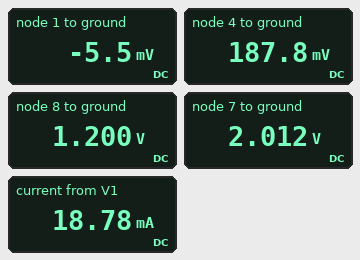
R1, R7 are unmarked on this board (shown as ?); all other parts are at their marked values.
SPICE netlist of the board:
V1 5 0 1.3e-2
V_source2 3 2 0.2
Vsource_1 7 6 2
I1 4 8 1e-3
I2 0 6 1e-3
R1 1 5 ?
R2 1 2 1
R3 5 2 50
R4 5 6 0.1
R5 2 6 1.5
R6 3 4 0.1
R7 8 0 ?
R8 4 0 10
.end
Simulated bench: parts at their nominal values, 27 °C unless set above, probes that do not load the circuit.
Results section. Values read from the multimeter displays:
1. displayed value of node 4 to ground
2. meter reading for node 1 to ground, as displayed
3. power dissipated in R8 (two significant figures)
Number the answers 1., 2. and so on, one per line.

1. 187.8 mV
2. -5.5 mV
3. 3.5 mW
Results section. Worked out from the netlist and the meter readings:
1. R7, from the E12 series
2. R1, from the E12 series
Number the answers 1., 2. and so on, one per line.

1. 1.2 kΩ
2. 3.9 Ω
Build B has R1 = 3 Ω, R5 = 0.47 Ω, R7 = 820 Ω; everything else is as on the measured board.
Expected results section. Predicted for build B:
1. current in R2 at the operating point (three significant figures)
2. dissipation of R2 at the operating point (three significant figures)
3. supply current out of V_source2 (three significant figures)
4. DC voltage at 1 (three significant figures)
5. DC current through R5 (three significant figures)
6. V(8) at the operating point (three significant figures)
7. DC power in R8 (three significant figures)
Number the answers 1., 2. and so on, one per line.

1. 2.58 mA
2. 6.65 µW
3. 21.1 mA
4. 5.26 mV
5. 18.3 mA
6. 820 mV
7. 4.02 mW
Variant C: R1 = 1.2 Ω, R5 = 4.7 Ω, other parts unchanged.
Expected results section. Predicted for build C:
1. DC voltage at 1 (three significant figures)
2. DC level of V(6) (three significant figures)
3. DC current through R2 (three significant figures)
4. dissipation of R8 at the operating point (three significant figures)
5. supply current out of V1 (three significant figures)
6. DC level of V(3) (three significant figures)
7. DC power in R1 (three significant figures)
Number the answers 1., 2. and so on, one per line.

1. -2.39 mV
2. 12.5 mV
3. 12.8 mA
4. 3.34 mW
5. 18.3 mA
6. 185 mV
7. 197 µW
